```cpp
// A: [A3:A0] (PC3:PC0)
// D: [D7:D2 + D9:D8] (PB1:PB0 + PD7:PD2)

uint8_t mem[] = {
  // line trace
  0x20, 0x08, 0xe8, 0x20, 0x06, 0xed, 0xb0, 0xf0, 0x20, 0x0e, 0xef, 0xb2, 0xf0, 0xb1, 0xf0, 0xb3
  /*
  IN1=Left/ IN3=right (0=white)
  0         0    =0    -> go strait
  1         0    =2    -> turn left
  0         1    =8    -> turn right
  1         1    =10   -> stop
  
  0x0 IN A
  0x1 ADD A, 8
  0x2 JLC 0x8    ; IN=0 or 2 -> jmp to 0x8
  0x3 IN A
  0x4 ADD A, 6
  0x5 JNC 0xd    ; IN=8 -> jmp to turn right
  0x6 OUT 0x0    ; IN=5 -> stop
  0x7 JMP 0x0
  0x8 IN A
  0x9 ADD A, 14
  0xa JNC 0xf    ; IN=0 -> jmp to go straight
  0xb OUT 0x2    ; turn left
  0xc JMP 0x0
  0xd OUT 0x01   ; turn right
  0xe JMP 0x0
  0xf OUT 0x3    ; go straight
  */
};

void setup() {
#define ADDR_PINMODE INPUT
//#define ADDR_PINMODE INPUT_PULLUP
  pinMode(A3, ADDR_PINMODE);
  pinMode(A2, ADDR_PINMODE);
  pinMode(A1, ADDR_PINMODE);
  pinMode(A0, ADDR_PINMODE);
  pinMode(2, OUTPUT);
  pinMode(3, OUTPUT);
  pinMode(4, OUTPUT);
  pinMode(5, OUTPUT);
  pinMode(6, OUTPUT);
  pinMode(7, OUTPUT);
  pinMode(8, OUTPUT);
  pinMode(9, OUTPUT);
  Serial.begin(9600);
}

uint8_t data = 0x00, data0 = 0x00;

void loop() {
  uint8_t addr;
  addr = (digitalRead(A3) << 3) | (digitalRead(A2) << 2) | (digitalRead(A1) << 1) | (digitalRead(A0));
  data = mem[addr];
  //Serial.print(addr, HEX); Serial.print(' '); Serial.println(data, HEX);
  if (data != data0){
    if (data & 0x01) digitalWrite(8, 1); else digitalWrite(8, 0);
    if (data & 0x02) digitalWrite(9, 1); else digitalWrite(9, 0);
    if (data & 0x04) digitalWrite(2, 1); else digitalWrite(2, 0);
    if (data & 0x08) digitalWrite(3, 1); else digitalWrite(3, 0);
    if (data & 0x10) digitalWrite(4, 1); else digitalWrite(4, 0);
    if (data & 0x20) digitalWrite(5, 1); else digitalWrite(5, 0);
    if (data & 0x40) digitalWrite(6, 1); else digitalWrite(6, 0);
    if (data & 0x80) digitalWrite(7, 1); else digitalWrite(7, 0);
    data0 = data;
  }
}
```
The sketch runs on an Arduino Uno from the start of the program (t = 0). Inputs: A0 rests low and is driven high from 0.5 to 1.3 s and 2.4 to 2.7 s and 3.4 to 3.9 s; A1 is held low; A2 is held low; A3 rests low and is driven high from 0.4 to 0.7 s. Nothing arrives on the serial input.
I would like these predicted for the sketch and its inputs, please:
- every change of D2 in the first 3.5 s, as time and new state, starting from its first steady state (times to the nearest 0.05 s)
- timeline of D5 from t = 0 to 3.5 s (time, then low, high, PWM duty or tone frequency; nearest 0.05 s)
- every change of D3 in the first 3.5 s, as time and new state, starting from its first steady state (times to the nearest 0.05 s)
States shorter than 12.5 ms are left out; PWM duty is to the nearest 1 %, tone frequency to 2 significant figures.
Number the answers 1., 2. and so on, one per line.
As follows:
1. 0 s low; 0.5 s high; 0.7 s low
2. 0 s high; 0.5 s low; 1.3 s high; 2.4 s low; 2.7 s high; 3.4 s low
3. 0 s low; 0.5 s high; 1.3 s low; 2.4 s high; 2.7 s low; 3.4 s high
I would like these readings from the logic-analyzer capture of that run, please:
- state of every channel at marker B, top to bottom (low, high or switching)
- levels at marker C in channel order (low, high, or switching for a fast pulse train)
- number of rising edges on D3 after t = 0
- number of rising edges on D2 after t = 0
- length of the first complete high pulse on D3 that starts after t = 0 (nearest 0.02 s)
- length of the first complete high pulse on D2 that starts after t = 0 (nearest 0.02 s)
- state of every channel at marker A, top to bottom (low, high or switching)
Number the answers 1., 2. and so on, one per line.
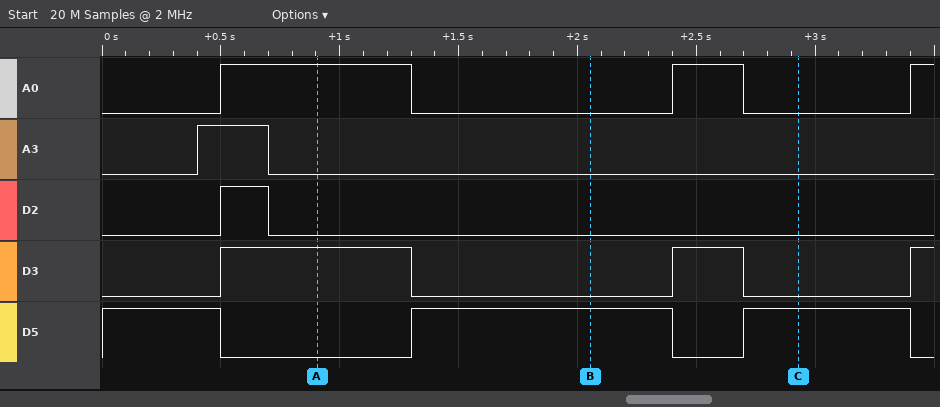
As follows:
1. A0 low, A3 low, D2 low, D3 low, D5 high
2. A0 low, A3 low, D2 low, D3 low, D5 high
3. 3
4. 1
5. 0.80 s
6. 0.20 s
7. A0 high, A3 low, D2 low, D3 high, D5 low
